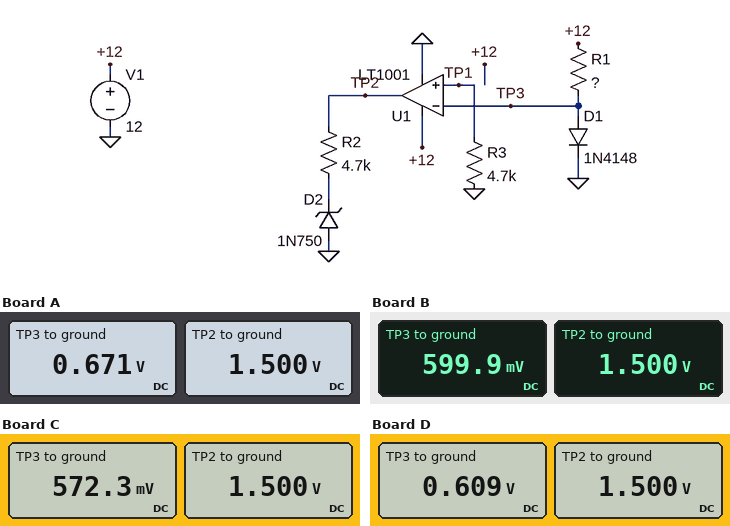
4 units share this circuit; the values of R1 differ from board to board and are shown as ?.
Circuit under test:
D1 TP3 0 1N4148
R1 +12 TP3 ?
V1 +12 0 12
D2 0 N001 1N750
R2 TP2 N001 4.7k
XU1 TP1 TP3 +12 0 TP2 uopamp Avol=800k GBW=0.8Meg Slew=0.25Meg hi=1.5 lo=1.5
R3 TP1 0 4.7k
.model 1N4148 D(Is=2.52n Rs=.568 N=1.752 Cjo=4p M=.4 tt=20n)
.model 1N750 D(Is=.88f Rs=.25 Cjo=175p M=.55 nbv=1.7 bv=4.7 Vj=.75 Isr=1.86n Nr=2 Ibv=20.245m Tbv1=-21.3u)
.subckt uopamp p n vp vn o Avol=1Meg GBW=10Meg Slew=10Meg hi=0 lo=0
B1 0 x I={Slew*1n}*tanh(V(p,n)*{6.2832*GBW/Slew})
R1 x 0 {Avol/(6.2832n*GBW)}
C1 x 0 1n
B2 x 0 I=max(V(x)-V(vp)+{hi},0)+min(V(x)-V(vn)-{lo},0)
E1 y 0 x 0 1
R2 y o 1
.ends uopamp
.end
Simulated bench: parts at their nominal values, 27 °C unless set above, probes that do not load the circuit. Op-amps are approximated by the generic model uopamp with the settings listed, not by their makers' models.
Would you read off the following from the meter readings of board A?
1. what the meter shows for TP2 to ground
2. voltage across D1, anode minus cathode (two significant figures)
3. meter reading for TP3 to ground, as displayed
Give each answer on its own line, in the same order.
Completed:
1.500 V
670 mV
0.671 V
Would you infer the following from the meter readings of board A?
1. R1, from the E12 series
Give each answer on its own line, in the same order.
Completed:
1.8 kΩ
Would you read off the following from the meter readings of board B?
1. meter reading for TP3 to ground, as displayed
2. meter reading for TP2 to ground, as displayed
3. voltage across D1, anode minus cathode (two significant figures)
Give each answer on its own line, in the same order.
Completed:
599.9 mV
1.500 V
600 mV
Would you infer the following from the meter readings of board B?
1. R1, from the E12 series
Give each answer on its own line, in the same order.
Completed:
8.2 kΩ
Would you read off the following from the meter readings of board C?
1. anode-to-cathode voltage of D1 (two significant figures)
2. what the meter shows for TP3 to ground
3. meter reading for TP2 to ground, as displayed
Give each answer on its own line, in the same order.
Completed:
570 mV
572.3 mV
1.500 V
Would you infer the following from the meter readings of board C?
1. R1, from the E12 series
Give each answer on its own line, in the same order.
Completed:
15 kΩ
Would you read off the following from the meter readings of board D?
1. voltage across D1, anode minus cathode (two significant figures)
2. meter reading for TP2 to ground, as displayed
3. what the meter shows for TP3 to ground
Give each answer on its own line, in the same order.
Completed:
610 mV
1.500 V
0.609 V
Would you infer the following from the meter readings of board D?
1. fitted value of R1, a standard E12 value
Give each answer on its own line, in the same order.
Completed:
6.8 kΩ
